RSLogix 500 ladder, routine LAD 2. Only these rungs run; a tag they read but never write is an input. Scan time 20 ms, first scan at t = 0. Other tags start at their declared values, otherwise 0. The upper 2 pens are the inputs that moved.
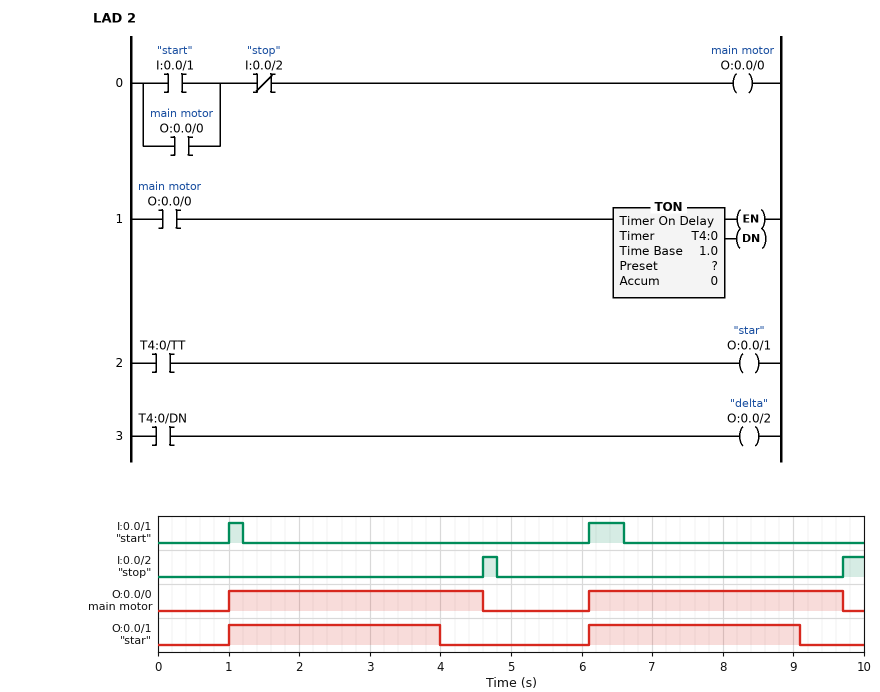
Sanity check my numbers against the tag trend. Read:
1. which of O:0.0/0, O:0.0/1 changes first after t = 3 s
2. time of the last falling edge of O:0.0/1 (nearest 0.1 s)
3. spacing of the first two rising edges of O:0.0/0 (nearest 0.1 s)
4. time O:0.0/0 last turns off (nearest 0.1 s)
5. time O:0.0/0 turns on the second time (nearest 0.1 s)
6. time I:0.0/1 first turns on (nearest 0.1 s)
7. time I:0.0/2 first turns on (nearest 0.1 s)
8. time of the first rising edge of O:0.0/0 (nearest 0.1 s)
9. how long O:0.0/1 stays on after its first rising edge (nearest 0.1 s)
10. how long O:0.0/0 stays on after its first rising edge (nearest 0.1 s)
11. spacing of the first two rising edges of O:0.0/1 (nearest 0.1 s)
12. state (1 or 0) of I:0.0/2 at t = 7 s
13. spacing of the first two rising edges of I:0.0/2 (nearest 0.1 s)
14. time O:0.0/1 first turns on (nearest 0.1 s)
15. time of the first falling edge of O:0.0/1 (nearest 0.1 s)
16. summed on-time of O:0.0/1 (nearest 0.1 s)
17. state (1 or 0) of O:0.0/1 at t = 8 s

O:0.0/1
9.1 s
5.1 s
9.7 s
6.1 s
1.0 s
4.6 s
1.0 s
3.0 s
3.6 s
5.1 s
0
5.1 s
1.0 s
4.0 s
6.0 s
1
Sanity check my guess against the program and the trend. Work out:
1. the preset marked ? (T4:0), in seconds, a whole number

3 s
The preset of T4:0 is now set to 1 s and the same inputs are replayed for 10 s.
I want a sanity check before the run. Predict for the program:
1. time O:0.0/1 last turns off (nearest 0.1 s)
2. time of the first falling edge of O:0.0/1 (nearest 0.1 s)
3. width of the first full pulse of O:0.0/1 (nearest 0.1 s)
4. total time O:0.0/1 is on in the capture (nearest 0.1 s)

7.1 s
2.0 s
1.0 s
2.0 s
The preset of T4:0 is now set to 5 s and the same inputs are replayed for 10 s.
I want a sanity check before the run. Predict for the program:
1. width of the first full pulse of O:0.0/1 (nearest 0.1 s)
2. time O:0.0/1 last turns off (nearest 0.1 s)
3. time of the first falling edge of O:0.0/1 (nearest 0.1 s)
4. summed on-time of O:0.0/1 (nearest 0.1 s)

3.6 s
9.7 s
4.6 s
7.2 s
